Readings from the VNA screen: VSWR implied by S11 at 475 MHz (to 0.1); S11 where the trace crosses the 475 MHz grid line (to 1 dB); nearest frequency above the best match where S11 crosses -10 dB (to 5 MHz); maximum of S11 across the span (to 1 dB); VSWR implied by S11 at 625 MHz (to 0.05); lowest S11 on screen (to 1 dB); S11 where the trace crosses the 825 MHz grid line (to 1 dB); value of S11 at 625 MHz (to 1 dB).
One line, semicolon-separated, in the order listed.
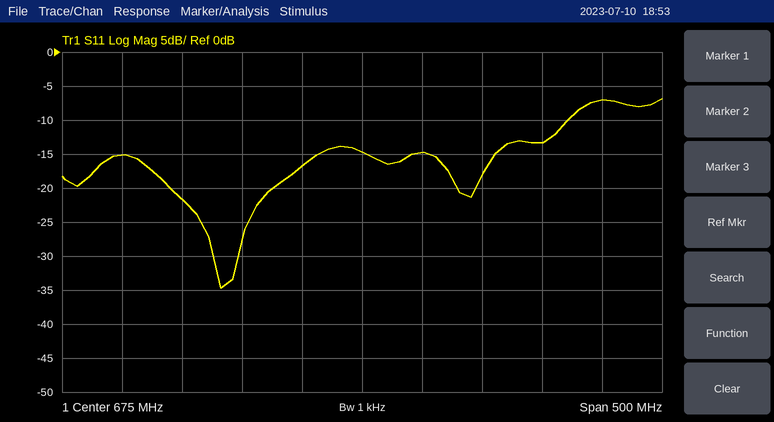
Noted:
1.4; -15 dB; 845 MHz; -7 dB; 1.35; -35 dB; -13 dB; -17 dB
